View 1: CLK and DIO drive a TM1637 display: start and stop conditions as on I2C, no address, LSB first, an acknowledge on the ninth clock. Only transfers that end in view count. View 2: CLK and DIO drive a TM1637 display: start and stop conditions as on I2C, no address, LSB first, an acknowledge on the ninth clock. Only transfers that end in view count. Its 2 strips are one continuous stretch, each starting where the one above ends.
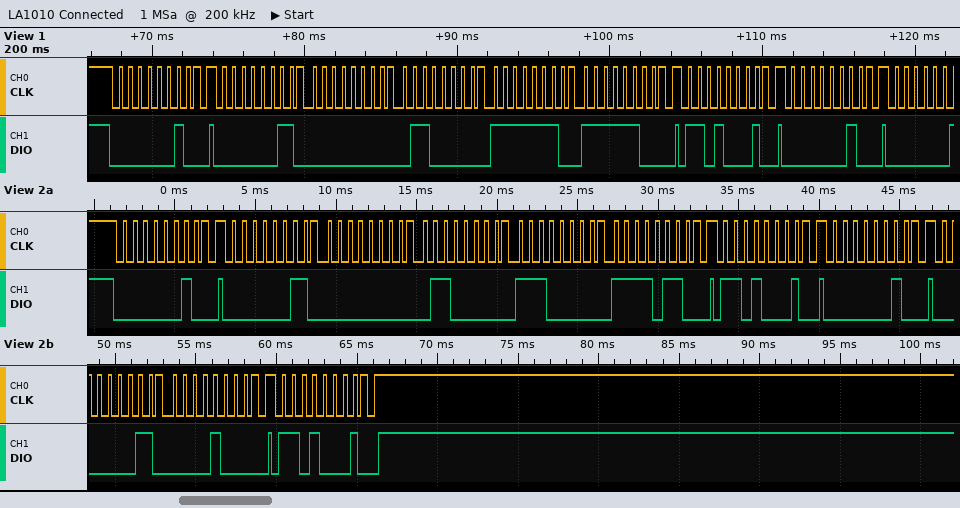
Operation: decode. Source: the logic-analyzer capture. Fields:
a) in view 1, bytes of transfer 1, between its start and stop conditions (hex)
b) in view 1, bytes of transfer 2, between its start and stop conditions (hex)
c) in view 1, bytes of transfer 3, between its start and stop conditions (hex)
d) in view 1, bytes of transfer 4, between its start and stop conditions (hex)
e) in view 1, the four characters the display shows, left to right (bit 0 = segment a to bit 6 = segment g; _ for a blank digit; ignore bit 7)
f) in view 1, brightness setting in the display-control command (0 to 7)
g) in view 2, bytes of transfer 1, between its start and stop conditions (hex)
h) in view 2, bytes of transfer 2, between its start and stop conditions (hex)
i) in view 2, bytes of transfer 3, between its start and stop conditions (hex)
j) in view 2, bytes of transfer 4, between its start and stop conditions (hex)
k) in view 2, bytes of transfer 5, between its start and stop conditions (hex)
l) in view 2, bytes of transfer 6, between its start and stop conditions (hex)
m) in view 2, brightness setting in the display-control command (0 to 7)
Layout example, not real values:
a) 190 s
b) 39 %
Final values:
a) 40
b) C0 00 06 7F 3F
c) 8B
d) 40
e) _180
f) 3
g) 40
h) C0 00 06 07 6F
i) 8B
j) 40
k) C0 10
l) 8B
m) 3
